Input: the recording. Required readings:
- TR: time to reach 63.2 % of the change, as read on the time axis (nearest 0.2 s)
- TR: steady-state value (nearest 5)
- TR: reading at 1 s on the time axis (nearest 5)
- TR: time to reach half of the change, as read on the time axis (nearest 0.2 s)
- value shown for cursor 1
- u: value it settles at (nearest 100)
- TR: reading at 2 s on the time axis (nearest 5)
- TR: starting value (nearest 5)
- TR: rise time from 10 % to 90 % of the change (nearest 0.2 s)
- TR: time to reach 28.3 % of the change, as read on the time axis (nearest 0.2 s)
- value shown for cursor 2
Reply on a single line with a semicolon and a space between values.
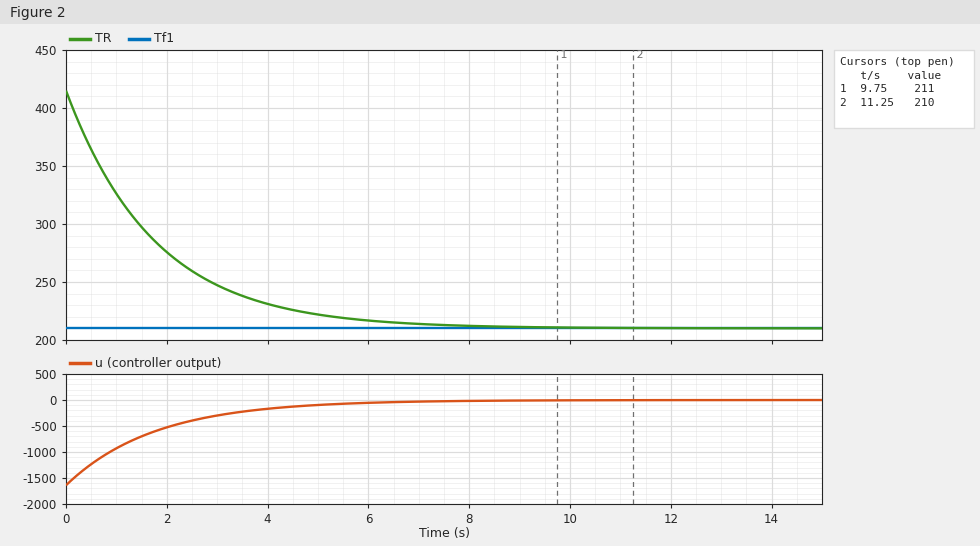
1.8 s; 210; 325; 1.2 s; 211; 0; 275; 415; 3.8 s; 0.6 s; 210
